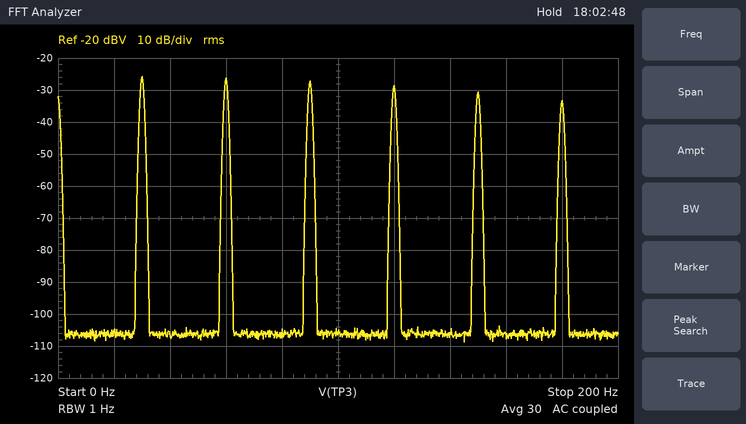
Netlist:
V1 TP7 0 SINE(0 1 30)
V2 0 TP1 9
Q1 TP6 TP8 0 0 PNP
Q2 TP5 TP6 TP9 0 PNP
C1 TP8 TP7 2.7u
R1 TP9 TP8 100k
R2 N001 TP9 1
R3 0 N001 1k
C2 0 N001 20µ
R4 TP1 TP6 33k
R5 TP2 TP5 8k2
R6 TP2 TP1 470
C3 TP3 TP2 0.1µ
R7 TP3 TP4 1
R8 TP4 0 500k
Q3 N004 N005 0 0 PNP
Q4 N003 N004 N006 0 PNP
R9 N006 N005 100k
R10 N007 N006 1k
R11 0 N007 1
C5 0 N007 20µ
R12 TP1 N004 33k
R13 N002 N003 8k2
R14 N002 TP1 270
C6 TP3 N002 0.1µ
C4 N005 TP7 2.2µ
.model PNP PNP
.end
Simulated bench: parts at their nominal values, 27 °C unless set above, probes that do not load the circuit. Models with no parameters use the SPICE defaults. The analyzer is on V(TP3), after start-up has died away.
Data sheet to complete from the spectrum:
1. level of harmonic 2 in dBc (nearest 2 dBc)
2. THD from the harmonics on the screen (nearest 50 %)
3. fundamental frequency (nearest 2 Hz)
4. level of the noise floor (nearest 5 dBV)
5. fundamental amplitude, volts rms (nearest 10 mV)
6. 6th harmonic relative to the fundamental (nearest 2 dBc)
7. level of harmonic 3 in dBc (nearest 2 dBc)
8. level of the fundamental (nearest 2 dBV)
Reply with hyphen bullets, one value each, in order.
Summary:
- 0 dBc
- 150 %
- 30 Hz
- -105 dBV
- 50 mV
- -8 dBc
- -2 dBc
- -26 dBV
